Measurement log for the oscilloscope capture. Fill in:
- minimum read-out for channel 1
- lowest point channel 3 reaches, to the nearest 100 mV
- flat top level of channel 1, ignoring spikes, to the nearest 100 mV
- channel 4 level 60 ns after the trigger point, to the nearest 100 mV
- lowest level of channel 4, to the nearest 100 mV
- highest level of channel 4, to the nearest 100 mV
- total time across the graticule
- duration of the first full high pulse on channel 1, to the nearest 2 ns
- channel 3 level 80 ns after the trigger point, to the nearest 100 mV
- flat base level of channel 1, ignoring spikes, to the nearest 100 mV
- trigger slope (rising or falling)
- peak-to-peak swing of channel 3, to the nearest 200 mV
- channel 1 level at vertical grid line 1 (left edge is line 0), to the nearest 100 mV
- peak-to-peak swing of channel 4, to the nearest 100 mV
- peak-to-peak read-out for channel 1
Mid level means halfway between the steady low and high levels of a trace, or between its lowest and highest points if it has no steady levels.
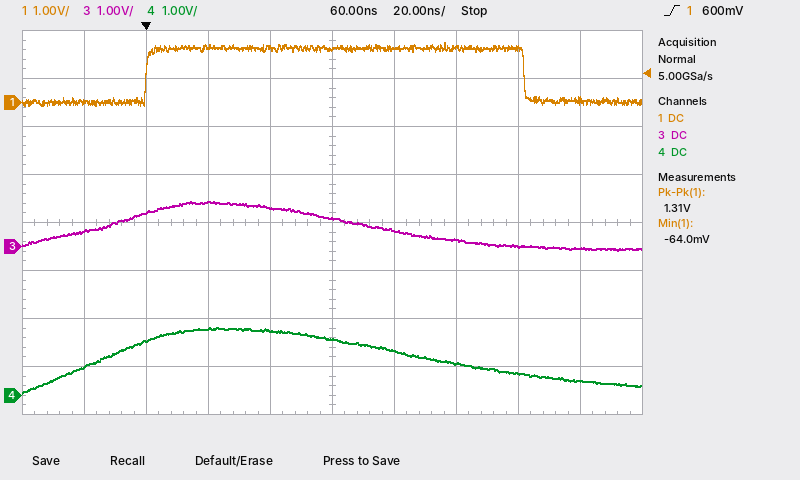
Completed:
-64.0 mV
-100 mV
1.1 V
1.2 V
0.0 V
1.4 V
200 ns
122 ns
300 mV
0.0 V
rising
1.0 V
0.0 V
1.4 V
1.31 V
